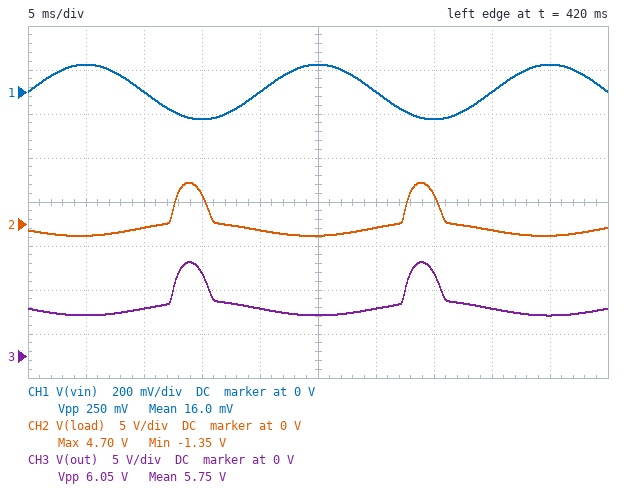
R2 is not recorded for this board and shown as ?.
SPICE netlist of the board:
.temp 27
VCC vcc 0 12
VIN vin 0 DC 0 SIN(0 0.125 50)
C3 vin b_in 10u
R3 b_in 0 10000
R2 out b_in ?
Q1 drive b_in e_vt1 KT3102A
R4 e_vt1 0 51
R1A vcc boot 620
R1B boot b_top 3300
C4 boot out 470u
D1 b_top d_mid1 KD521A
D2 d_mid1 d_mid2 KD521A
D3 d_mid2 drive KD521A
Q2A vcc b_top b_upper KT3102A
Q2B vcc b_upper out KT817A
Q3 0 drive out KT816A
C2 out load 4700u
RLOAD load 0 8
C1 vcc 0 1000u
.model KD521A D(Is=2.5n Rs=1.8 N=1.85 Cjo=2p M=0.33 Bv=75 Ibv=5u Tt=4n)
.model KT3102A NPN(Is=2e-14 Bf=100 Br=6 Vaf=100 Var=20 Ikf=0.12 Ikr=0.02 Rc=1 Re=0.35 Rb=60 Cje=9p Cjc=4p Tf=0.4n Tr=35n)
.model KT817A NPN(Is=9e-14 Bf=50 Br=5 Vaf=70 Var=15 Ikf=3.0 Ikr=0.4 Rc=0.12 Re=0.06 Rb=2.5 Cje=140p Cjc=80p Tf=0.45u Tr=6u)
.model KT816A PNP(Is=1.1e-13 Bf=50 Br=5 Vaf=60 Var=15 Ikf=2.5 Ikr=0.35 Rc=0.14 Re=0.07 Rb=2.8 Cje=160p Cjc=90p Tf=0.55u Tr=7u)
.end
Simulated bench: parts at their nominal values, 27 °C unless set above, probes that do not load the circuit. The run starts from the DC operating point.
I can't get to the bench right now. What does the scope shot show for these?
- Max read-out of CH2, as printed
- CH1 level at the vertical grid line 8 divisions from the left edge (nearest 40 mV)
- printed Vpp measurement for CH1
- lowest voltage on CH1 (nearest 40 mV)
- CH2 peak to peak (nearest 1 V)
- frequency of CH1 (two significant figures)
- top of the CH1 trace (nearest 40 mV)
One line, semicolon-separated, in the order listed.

4.70 V; 0 V; 250 mV; -120 mV; 6 V; 50 Hz; 120 mV
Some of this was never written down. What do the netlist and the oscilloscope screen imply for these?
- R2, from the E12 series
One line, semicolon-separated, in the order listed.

47 kΩ
